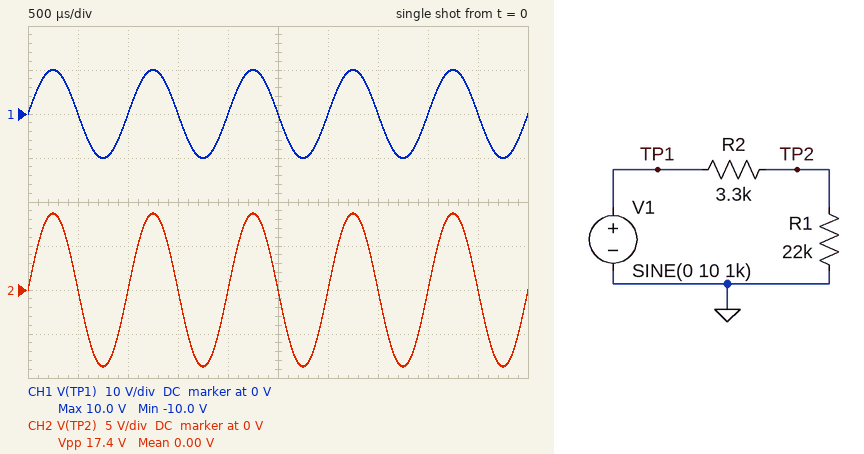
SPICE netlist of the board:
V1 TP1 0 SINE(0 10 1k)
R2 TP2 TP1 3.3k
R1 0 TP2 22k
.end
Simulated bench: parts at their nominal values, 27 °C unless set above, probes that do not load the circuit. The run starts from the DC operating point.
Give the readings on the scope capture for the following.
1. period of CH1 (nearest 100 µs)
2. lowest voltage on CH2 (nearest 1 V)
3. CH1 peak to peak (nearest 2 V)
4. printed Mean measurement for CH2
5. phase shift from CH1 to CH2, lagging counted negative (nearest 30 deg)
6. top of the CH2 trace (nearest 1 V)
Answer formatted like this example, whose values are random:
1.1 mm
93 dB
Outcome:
1.0 ms
-9 V
20 V
0.00 V
0 deg
9 V
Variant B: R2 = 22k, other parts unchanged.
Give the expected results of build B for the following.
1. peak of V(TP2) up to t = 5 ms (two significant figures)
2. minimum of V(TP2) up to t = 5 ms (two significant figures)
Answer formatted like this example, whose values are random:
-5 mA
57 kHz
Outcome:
5.0 V
-5.0 V
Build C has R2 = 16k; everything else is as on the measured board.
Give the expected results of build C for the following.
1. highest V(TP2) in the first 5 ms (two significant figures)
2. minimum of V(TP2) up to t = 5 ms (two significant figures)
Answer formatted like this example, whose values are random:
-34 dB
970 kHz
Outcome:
5.8 V
-5.8 V
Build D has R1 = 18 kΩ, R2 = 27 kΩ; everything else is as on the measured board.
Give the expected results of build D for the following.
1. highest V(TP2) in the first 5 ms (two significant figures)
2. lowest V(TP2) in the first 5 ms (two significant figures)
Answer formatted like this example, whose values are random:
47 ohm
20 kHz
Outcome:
4.0 V
-4.0 V
